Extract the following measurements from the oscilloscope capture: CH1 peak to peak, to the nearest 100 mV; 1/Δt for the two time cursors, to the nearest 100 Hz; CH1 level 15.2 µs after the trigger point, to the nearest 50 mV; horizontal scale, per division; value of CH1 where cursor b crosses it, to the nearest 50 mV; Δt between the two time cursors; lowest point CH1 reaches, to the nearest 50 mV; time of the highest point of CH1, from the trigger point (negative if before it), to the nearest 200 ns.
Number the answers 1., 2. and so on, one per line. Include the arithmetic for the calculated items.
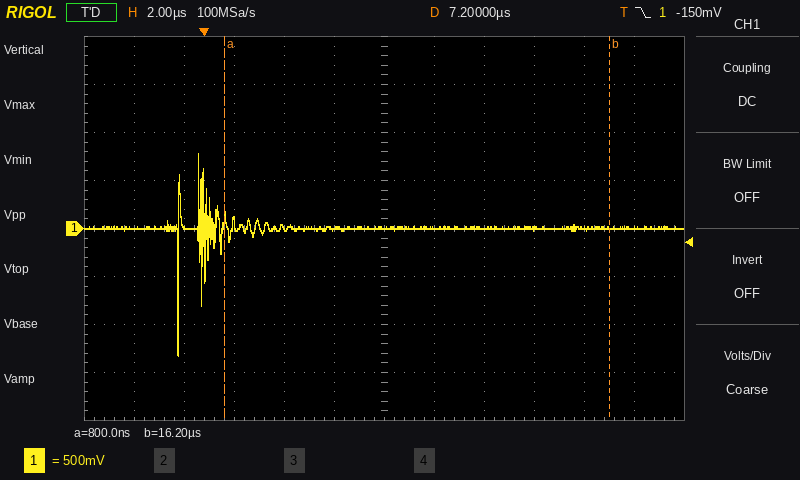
1. 2.10 V
2. 1 / 15.4 µs ≈ 64.9 kHz
3. 0 mV
4. 2 µs
5. 0 mV
6. 16.2 µs − (800 ns) = 15.4 µs
7. -1.30 V
8. -200 ns
